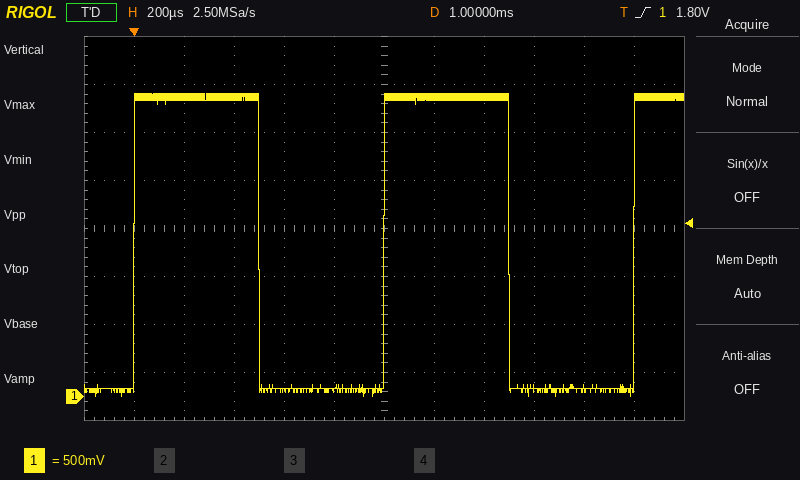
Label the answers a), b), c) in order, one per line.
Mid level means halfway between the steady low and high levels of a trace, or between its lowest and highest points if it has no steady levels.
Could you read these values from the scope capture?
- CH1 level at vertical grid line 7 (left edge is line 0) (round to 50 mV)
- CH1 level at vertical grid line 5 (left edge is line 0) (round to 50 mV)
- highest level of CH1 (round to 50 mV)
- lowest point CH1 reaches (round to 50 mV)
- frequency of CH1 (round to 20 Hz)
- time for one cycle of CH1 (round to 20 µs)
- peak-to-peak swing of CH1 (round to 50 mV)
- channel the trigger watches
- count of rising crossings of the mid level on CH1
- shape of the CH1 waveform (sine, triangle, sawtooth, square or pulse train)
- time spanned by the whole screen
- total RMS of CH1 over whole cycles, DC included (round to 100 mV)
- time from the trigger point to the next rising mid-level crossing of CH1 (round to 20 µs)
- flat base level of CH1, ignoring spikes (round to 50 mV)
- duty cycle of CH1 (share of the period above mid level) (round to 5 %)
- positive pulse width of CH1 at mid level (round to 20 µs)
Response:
a) 3.10 V
b) 100 mV
c) 3.15 V
d) 0 mV
e) 1.00 kHz
f) 1.00 ms
g) 3.15 V
h) CH1
i) 3
j) square
k) 2.4 ms
l) 2.2 V
m) 1.00 ms
n) 100 mV
o) 50 %
p) 500 µs
